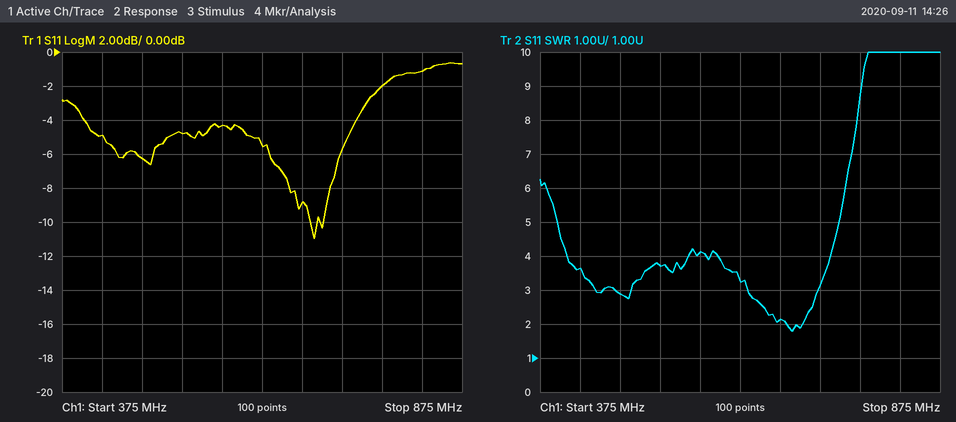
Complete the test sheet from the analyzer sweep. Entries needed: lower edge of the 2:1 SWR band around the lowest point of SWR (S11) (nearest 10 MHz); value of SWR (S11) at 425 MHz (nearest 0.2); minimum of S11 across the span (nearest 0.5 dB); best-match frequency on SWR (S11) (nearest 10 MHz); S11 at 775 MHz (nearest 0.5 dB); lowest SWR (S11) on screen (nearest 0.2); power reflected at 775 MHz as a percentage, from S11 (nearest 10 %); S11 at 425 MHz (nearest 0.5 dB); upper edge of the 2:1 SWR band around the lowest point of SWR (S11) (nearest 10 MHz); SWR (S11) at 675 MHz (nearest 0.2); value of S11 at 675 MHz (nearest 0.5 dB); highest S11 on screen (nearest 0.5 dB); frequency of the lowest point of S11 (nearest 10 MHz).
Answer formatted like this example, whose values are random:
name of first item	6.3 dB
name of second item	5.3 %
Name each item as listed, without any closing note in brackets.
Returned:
lower edge of the 2:1 SWR band around the lowest point of SWR (S11)	680 MHz
value of SWR (S11) at 425 MHz	3.6
minimum of S11 across the span	-11.0 dB
best-match frequency on SWR (S11)	690 MHz
S11 at 775 MHz	-2.0 dB
lowest SWR (S11) on screen	1.8
power reflected at 775 MHz as a percentage, from S11	60 %
S11 at 425 MHz	-5.0 dB
upper edge of the 2:1 SWR band around the lowest point of SWR (S11)	700 MHz
SWR (S11) at 675 MHz	2.2
value of S11 at 675 MHz	-9.0 dB
highest S11 on screen	-0.5 dB
frequency of the lowest point of S11	690 MHz
